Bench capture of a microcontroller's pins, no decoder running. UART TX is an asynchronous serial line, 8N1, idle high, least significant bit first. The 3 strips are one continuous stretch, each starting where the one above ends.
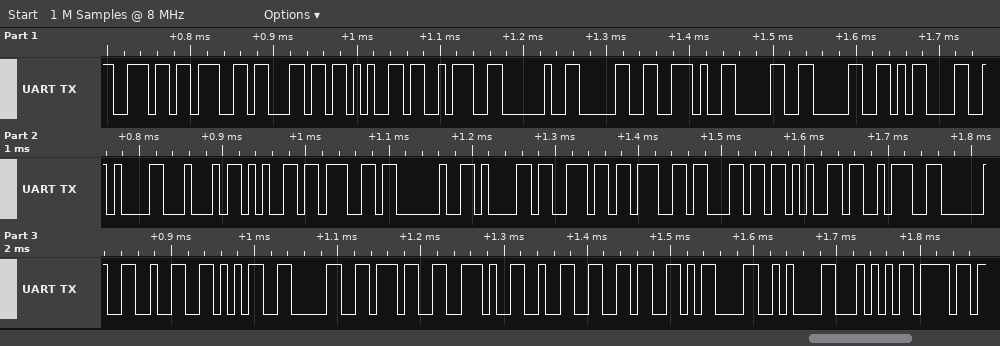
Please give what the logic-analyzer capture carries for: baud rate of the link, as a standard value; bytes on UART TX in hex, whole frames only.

115200 baud
6E 67 6C 65 3A 20 30 2E 30 30 0D 0A 44 65 67 20 61 6E 67 6C 65 3A 20 32 35 30 37 2E 32 36 0D 0A 54 6F
